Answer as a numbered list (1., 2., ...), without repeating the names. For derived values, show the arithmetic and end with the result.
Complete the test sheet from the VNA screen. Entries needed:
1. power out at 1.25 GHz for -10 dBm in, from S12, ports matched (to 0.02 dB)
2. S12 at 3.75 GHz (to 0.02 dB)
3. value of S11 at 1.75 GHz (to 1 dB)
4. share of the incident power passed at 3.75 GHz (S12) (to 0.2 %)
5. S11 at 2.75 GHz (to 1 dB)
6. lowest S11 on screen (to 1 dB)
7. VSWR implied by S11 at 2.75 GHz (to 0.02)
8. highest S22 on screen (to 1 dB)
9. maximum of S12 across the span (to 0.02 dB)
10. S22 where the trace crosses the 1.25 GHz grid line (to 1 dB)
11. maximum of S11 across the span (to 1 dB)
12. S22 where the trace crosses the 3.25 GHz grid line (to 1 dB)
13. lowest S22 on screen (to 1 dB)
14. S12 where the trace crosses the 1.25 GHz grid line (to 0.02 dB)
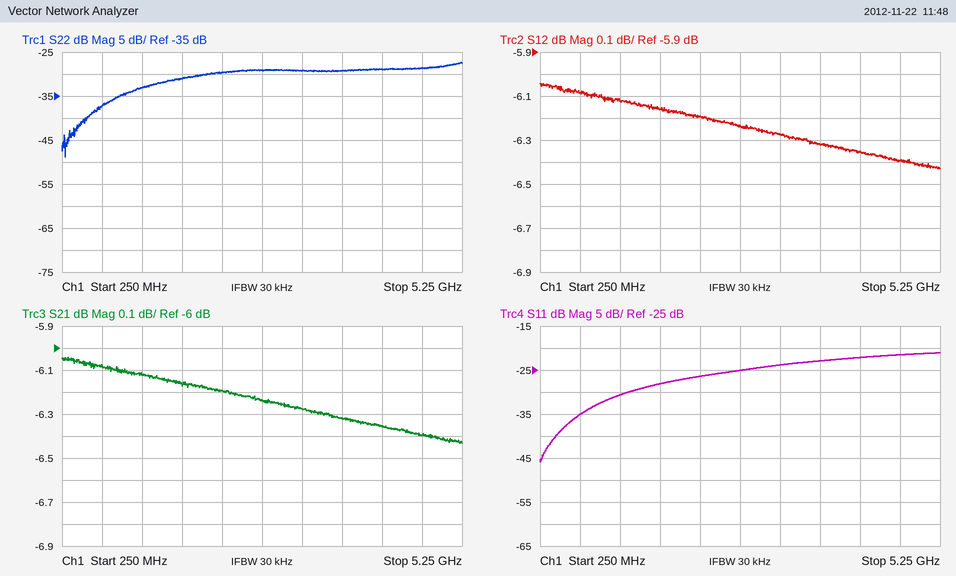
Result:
1. -10 dBm + (-6.12 dB) = -16.12 dBm
2. -6.32 dB
3. -28 dB
4. 10^(-6.32/10) ≈ 23.3 %, so 23.4 % to the nearest 0.2 %
5. -25 dB
6. -46 dB
7. |Γ| = 10^(-25/20) = 0.0562; VSWR = (1 + 0.0562)/(1 − 0.0562) ≈ 1.12
8. -27 dB
9. -6.04 dB
10. -33 dB
11. -21 dB
12. -29 dB
13. -49 dB
14. -6.12 dB
